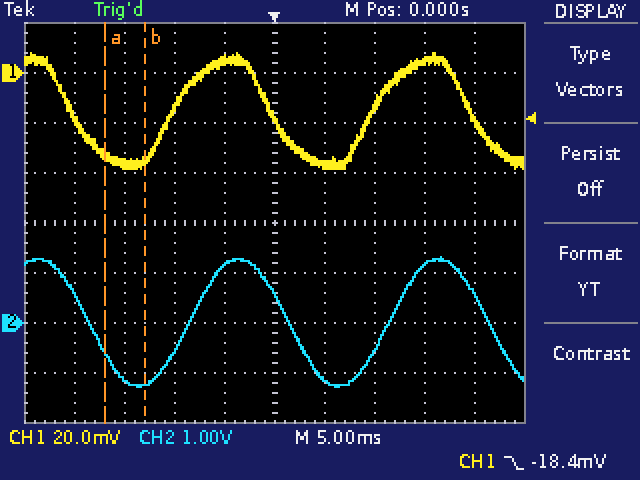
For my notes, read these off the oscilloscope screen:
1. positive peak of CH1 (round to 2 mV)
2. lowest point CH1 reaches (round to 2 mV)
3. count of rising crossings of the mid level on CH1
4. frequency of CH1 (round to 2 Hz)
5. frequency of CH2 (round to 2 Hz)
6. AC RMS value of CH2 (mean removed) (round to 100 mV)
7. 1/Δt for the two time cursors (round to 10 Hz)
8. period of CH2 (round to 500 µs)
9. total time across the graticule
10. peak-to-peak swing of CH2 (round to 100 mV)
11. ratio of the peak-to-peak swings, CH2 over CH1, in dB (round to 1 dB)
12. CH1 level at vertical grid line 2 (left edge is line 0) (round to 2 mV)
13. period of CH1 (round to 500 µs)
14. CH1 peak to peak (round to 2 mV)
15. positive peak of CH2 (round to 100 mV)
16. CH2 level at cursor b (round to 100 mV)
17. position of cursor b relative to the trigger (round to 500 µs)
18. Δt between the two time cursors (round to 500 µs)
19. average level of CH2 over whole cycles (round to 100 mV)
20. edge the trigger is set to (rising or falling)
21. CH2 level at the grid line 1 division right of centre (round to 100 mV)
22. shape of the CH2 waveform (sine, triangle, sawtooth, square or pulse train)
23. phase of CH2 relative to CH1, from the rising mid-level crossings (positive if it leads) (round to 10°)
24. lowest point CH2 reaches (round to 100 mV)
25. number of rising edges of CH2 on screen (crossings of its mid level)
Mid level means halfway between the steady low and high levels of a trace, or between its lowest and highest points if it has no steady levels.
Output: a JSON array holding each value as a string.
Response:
["8 mV", "-38 mV", "2", "50 Hz", "50 Hz", "900 mV", "250 Hz", "20.0 ms", "50 ms", "2.6 V", "35 dB", "-36 mV", "20.0 ms", "46 mV", "1.3 V", "-1.2 V", "-13.0 ms", "4.0 ms", "0.0 V", "falling", "-1.1 V", "sine", "-30°", "-1.3 V", "2"]
